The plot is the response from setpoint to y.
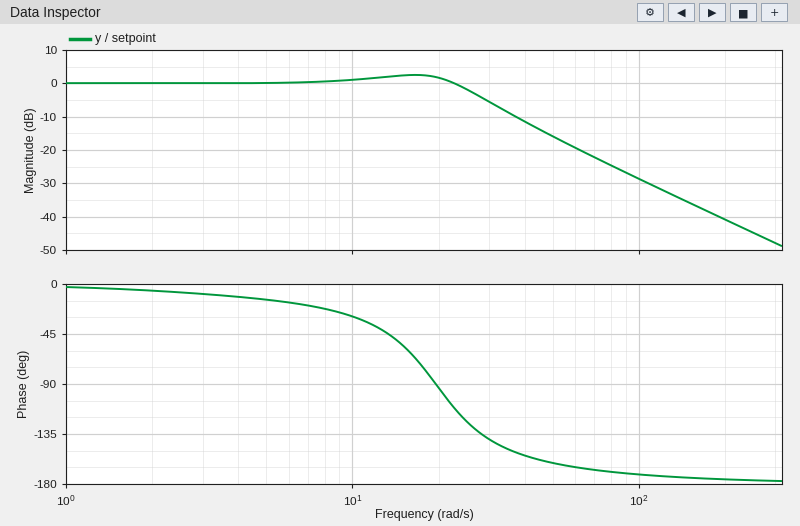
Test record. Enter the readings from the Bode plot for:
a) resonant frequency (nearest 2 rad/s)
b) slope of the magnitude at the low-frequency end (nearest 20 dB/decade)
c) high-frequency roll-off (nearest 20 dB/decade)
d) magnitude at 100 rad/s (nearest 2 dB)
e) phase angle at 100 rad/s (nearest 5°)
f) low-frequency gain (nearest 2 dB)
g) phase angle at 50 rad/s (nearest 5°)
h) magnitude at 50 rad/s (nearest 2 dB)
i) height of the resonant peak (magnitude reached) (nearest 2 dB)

16 rad/s
0 dB/decade
-40 dB/decade
-28 dB
-170°
0 dB
-160°
-16 dB
2 dB
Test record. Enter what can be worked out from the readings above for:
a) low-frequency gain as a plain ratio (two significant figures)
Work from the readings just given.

1.0
